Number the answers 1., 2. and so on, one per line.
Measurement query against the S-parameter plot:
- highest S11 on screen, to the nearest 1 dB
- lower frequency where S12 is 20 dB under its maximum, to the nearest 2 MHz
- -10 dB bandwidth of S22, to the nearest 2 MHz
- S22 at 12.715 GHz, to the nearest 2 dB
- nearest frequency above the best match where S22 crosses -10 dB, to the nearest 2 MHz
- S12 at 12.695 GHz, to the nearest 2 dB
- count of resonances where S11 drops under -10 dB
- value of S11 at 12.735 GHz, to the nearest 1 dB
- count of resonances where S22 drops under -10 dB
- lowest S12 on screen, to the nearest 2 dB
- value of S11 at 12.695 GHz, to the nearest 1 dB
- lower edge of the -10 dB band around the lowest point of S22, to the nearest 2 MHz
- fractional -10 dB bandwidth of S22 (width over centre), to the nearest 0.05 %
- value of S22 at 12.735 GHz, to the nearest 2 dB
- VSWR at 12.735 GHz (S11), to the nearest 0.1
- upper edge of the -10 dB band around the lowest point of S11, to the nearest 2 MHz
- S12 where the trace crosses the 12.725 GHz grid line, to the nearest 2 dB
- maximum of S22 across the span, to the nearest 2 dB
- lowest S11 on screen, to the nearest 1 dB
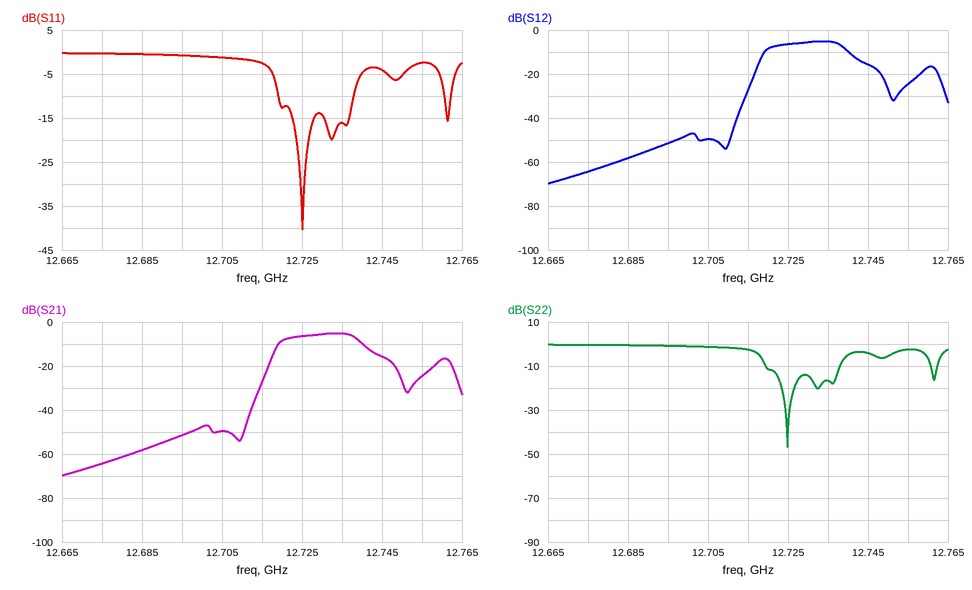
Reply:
1. 0 dB
2. 12.716 GHz
3. 18 MHz
4. -2 dB
5. 12.738 GHz
6. -52 dB
7. 3
8. -16 dB
9. 3
10. -70 dB
11. -1 dB
12. 12.720 GHz
13. 0.15 %
14. -16 dB
15. 1.4
16. 12.738 GHz
17. -6 dB
18. 0 dB
19. -40 dB
